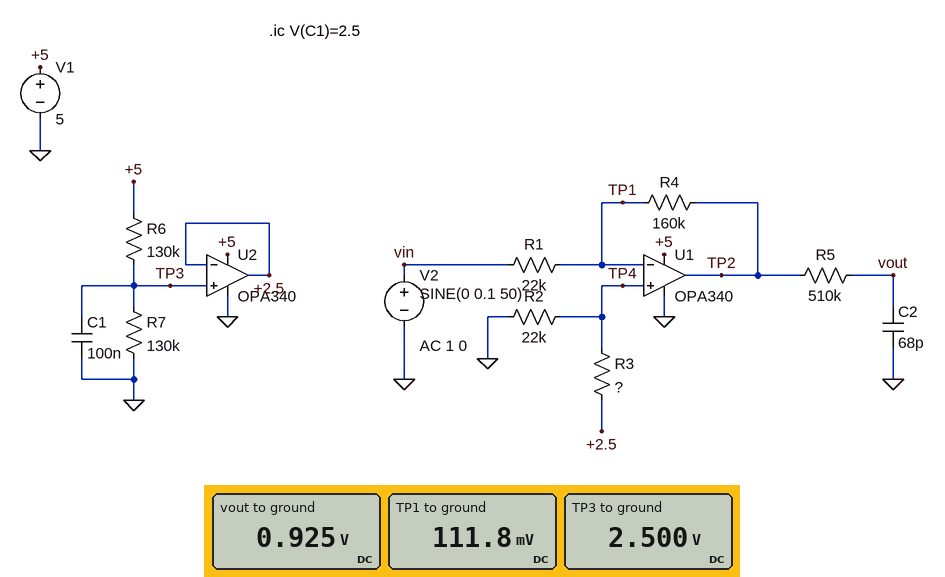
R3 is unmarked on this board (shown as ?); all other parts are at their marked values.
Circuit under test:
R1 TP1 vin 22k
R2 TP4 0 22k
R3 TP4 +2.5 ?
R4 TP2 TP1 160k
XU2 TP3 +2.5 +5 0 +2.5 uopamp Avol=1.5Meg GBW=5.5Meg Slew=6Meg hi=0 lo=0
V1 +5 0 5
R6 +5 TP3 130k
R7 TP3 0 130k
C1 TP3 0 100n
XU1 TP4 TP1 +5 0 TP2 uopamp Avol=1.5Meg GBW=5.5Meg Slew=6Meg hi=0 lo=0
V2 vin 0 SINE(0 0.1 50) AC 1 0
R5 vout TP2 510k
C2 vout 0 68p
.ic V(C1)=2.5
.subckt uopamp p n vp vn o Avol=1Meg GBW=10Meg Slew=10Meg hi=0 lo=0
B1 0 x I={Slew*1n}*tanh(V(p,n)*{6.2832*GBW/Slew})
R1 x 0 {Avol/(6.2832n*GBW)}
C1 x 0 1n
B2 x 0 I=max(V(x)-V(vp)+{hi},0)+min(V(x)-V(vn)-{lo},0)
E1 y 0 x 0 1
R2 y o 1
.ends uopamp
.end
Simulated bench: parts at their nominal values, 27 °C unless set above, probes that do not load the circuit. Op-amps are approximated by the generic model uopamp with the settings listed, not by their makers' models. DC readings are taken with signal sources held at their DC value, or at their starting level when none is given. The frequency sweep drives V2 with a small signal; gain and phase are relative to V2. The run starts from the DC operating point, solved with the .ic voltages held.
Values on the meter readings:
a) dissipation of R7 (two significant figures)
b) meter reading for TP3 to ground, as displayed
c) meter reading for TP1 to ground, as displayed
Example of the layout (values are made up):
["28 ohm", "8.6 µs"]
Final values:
["48 µW", "2.500 V", "111.8 mV"]
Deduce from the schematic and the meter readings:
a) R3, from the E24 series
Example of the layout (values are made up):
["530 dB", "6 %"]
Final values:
["470 kΩ"]
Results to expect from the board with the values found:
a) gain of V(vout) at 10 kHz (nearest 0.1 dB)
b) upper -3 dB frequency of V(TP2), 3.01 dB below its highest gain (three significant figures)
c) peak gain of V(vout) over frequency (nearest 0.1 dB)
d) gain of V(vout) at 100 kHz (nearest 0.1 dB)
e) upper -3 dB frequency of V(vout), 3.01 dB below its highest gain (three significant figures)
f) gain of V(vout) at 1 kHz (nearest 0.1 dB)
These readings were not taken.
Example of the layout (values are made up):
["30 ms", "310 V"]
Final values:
["9.6 dB", "665 kHz", "17.2 dB", "-9.6 dB", "4.59 kHz", "17.0 dB"]
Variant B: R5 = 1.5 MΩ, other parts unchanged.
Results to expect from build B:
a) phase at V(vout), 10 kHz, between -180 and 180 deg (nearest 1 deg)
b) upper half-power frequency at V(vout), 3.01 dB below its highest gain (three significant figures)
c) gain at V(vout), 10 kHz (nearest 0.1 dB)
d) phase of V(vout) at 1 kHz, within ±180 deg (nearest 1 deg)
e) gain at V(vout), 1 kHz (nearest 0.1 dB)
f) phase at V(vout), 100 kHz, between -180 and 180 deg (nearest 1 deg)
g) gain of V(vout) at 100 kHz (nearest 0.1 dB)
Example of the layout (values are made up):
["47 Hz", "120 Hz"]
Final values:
["98 deg", "1.56 kHz", "1.0 dB", "147 deg", "15.7 dB", "82 deg", "-19.0 dB"]
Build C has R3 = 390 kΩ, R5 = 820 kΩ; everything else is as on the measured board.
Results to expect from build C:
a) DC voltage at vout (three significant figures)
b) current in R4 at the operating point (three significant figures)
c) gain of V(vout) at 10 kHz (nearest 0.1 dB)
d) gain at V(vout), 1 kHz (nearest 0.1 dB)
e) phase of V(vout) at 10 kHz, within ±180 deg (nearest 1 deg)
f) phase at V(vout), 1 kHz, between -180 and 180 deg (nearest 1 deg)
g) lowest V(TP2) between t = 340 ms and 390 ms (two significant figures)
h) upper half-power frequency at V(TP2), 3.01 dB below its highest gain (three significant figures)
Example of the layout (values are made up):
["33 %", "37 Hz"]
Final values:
["1.10 V", "6.07 µA", "6.0 dB", "16.7 dB", "105 deg", "161 deg", "380 mV", "665 kHz"]
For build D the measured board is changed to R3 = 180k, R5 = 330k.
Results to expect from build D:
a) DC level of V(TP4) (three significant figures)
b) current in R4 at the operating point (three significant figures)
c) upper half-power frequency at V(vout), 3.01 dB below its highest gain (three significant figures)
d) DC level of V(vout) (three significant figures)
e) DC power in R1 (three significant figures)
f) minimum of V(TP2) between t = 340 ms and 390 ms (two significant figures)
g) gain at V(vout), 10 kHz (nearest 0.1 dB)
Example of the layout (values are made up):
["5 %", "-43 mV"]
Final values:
["272 mV", "12.4 µA", "7.09 kHz", "2.25 V", "3.37 µW", "1.5 V", "12.5 dB"]
